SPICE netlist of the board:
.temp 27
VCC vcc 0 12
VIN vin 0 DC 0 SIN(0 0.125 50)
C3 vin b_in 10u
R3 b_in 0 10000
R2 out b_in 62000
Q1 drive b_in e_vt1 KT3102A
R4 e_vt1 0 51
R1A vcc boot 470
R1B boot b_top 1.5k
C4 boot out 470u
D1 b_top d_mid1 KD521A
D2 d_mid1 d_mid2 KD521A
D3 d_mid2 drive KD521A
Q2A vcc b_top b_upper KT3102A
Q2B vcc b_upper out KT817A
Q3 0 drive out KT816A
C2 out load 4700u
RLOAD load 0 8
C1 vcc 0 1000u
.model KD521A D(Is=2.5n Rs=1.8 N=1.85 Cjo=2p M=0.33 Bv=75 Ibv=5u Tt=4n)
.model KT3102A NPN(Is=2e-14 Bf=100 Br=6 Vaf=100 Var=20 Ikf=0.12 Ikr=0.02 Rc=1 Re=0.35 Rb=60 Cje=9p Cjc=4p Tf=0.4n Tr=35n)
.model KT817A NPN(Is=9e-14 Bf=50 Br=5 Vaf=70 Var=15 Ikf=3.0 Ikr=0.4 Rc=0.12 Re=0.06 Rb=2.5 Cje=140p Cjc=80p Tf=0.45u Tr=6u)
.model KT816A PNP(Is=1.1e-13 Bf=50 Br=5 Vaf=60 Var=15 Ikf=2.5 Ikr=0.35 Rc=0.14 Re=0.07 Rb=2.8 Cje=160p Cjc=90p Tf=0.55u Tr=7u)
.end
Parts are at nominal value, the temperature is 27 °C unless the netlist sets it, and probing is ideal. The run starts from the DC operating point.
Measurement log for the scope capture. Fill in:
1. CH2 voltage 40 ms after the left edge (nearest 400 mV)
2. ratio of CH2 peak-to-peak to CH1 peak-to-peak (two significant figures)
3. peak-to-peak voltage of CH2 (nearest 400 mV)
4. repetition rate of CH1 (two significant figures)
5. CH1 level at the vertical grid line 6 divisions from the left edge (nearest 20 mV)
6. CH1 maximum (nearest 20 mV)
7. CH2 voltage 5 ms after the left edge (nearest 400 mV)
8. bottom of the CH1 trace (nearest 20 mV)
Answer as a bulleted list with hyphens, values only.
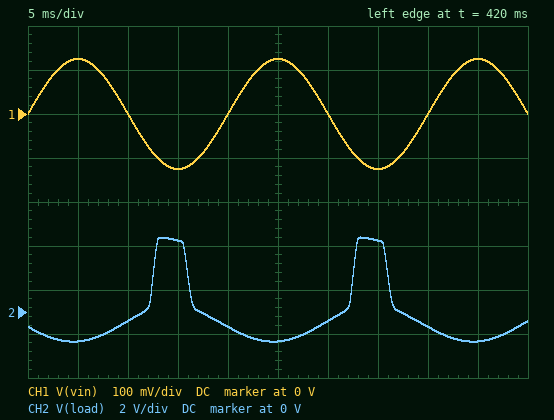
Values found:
- -800 mV
- 19
- 4.8 V
- 50 Hz
- 0 V
- 120 mV
- -1.2 V
- -120 mV
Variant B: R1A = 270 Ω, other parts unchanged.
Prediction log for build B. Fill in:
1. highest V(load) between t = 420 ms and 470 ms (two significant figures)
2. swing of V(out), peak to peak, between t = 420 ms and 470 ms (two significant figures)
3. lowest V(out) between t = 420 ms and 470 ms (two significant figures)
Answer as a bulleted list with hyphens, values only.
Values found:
- 3.3 V
- 4.6 V
- 6.5 V
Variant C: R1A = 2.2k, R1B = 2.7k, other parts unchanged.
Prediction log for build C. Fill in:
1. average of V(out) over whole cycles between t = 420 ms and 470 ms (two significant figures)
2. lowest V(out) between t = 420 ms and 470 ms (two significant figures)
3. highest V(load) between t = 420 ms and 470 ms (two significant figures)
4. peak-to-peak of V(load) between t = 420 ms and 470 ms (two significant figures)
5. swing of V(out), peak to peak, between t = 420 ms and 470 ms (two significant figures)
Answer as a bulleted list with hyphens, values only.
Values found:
- 7.0 V
- 5.7 V
- 4.0 V
- 5.4 V
- 5.3 V
